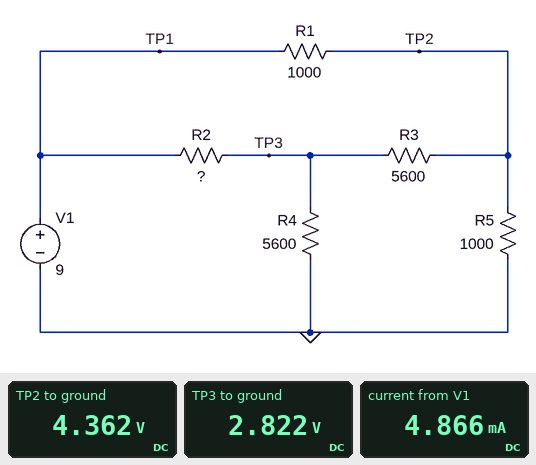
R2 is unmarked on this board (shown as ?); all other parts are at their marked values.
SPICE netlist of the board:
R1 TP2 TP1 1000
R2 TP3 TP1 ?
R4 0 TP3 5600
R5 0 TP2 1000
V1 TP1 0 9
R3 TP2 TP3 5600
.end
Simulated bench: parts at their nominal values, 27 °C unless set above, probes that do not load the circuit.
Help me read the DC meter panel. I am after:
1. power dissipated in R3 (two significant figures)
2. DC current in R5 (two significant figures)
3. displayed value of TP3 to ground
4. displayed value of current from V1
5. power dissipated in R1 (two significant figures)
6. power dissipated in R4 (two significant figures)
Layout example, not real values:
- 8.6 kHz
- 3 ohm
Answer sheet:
- 420 µW
- 4.4 mA
- 2.822 V
- 4.866 mA
- 22 mW
- 1.4 mW
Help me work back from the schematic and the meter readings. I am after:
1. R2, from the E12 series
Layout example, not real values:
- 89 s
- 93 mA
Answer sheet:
- 27 kΩ
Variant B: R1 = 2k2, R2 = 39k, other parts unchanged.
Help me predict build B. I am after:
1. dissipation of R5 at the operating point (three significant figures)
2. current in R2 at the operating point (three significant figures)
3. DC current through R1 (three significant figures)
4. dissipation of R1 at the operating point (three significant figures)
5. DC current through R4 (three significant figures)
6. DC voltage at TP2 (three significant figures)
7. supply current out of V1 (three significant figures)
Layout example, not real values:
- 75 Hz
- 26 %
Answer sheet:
- 7.34 mW
- 183 µA
- 2.86 mA
- 18.0 mW
- 333 µA
- 2.71 V
- 3.04 mA
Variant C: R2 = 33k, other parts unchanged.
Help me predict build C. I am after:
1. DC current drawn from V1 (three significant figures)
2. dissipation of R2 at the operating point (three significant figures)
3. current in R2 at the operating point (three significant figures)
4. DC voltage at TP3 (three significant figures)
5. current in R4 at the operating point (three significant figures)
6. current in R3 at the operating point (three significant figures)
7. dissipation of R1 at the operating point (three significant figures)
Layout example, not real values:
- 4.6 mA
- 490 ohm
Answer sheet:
- 4.84 mA
- 1.20 mW
- 191 µA
- 2.71 V
- 484 µA
- 293 µA
- 21.6 mW
